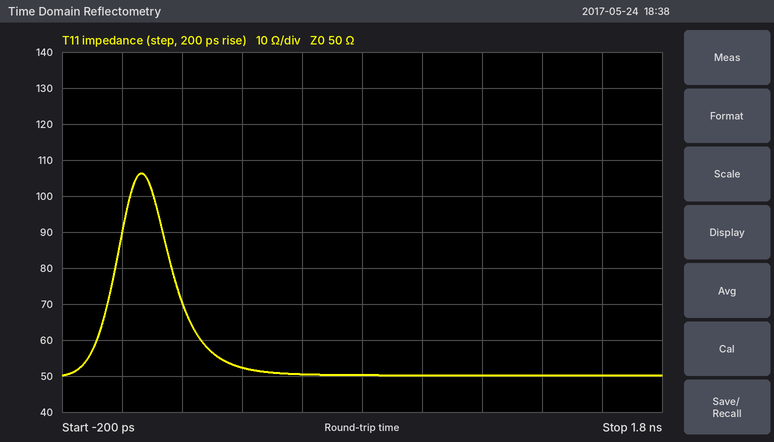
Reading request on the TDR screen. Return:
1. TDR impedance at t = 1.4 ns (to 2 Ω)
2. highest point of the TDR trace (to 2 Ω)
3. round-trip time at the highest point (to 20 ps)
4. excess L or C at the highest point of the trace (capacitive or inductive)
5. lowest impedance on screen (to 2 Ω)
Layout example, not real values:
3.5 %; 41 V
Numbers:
50 Ω; 106 Ω; 60 ps; inductive; 50 Ω
